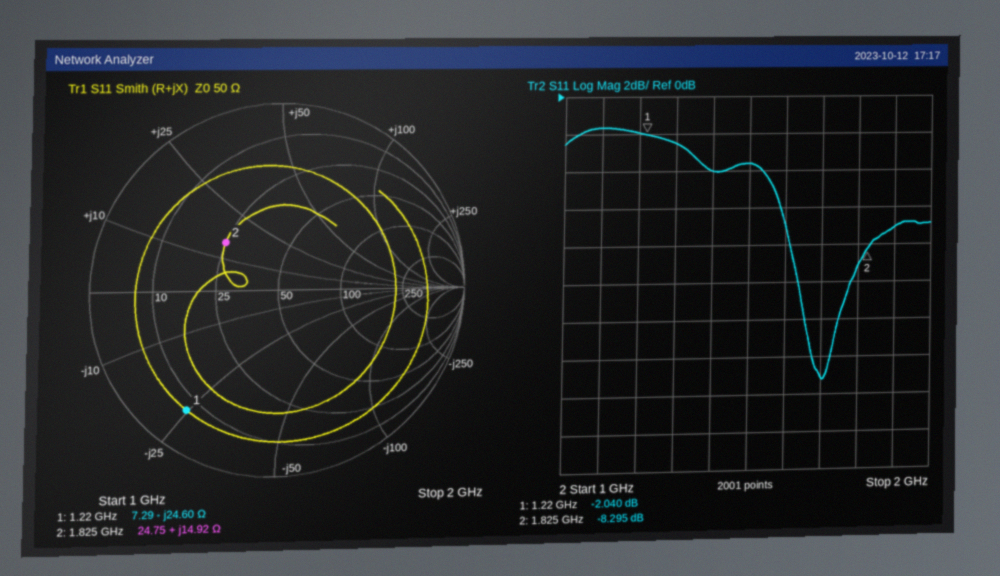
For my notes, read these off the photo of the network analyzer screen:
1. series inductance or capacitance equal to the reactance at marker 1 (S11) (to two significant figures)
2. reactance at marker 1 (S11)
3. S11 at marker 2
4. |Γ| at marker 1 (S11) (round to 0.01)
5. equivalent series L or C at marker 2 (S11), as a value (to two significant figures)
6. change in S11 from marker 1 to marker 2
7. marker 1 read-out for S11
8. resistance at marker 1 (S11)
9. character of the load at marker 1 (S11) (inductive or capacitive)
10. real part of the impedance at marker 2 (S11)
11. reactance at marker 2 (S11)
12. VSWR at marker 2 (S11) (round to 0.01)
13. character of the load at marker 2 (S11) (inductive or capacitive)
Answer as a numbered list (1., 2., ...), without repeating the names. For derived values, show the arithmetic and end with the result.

1. C = 1/(2π × 1.22 GHz × 24.6 Ω) ≈ 5.3 pF
2. -24.60 Ω
3. -8.295 dB
4. 0.79
5. L = 14.92 Ω/(2π × 1.825 GHz) ≈ 1.3 nH
6. -8.295 − (-2.04) = -6.255 dB
7. -2.040 dB
8. 7.29 Ω
9. capacitive
10. 24.75 Ω
11. +14.92 Ω
12. (1 + 0.3848)/(1 − 0.3848) ≈ 2.25
13. inductive
